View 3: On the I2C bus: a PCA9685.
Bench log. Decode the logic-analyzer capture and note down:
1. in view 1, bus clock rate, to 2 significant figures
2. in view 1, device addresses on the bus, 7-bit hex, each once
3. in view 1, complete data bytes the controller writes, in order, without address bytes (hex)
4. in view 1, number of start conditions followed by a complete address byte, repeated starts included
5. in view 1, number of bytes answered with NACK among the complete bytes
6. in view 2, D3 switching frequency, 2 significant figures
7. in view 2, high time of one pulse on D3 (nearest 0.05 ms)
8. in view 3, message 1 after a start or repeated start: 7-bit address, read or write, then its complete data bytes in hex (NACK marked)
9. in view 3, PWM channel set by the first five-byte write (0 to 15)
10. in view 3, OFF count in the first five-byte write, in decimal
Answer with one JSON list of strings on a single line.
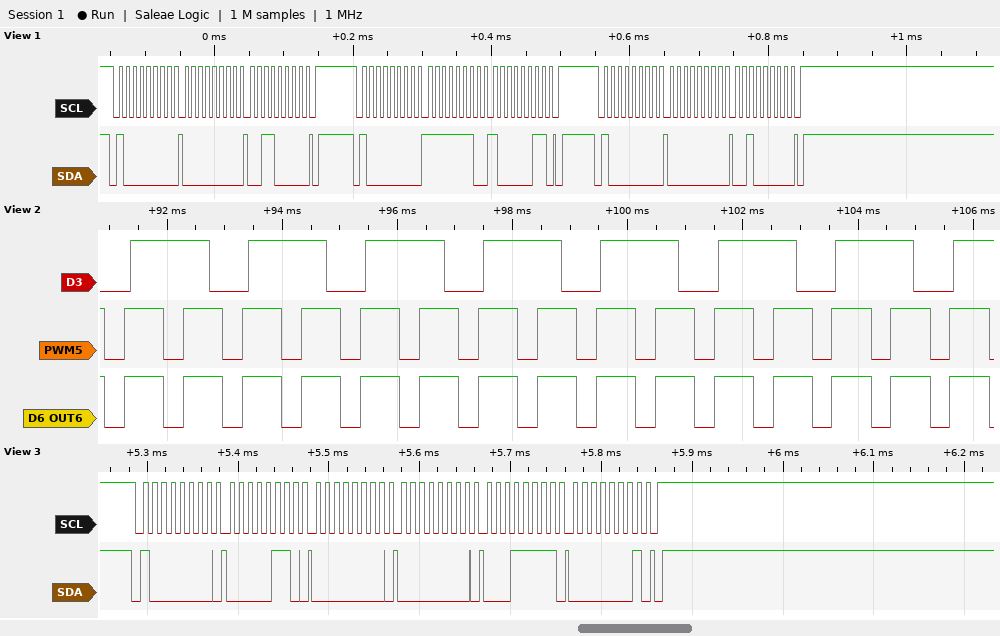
["100 kHz", "0x40", "00 30 FE 83 00 20", "3", "0", "490 Hz", "1.35 ms", "0x40 write: 06 00 00 1F 01", "0", "287"]
